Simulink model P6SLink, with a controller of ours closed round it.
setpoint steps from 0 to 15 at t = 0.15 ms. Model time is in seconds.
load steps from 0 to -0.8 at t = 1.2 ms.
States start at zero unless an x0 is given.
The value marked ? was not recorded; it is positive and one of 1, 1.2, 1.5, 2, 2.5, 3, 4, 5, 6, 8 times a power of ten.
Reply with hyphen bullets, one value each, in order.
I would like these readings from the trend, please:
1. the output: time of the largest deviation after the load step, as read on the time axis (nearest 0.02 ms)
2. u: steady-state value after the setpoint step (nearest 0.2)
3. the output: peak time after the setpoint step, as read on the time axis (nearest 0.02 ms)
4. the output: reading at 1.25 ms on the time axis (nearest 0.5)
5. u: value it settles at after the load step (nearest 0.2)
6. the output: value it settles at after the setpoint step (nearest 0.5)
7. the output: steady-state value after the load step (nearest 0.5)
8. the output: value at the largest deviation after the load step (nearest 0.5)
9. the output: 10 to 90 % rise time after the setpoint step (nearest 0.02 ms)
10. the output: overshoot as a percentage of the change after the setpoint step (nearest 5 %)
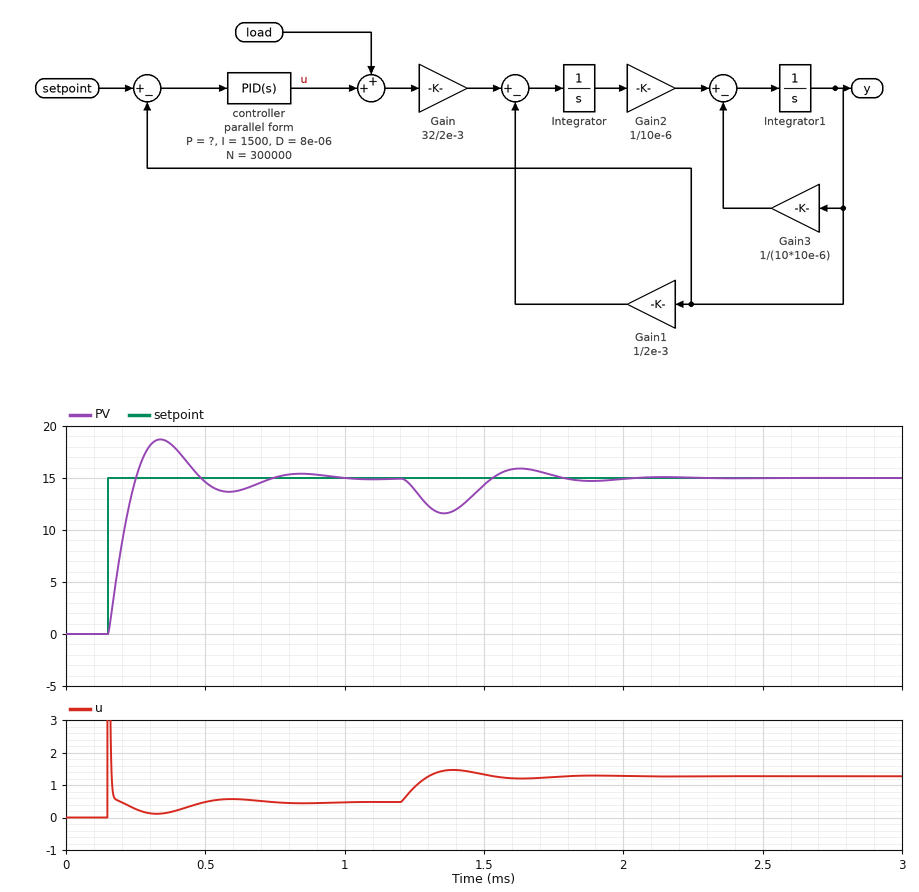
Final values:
- 1.36 ms
- 0.4
- 0.34 ms
- 14.0
- 1.2
- 15.0
- 15.0
- 11.5
- 0.08 ms
- 25 %
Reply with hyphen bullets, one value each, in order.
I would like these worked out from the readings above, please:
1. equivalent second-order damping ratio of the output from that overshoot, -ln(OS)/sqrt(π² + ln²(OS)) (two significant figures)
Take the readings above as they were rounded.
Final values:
- 0.40
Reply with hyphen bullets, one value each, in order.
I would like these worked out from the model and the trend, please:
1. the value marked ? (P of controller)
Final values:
- 0.15
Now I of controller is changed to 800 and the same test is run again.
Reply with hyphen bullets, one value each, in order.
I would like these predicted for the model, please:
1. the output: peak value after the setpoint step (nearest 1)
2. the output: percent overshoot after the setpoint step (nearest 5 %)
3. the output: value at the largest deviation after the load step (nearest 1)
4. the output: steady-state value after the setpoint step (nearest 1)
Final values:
- 17
- 10 %
- 11
- 15
